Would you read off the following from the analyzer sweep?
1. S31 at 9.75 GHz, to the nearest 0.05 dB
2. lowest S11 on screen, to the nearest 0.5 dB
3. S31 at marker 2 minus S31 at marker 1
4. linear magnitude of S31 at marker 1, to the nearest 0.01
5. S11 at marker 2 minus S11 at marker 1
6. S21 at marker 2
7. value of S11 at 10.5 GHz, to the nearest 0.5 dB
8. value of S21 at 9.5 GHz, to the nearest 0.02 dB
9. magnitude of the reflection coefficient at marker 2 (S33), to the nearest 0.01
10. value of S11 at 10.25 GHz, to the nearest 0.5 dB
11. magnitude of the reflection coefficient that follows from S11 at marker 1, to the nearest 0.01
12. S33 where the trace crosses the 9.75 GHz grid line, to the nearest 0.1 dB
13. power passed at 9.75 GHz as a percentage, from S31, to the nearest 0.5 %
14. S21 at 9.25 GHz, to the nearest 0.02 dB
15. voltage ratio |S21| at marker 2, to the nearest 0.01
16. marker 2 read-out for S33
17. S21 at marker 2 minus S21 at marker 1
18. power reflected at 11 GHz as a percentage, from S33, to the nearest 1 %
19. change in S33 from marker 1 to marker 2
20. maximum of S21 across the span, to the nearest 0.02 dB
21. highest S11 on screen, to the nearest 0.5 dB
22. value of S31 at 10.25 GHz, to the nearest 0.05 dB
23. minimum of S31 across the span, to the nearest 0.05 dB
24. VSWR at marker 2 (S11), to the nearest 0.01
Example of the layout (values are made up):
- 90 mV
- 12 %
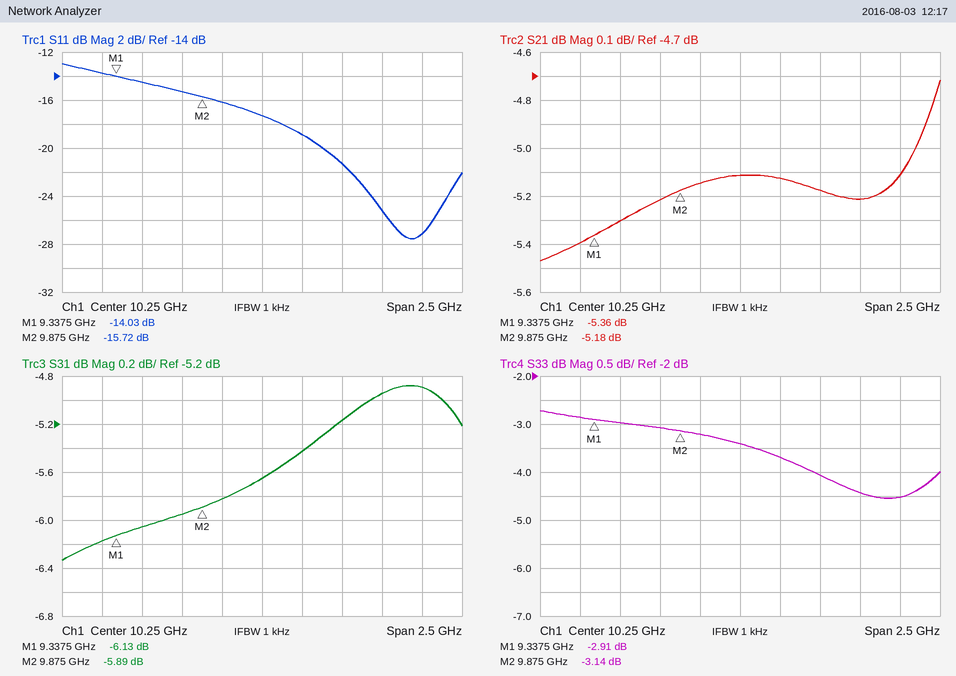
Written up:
- -5.95 dB
- -27.5 dB
- 0.24 dB
- 0.49
- -1.69 dB
- -5.18 dB
- -19.0 dB
- -5.30 dB
- 0.70
- -17.5 dB
- 0.20
- -3.1 dB
- 25.5 %
- -5.40 dB
- 0.55
- -3.14 dB
- 0.18 dB
- 36 %
- -0.23 dB
- -4.72 dB
- -13.0 dB
- -5.65 dB
- -6.35 dB
- 1.39
